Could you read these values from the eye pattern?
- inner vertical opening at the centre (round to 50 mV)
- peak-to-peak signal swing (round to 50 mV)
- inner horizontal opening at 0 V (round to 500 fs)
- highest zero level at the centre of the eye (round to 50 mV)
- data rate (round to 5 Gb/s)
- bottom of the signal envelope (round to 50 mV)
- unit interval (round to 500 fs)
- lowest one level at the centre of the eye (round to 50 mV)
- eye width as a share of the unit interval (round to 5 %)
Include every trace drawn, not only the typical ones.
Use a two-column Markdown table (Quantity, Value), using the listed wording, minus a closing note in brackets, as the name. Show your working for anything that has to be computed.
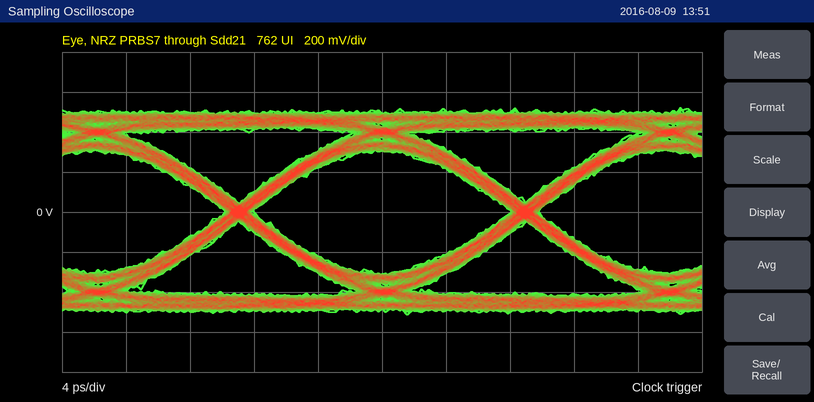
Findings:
| Quantity | Value |
|---|---|
| inner vertical opening at the centre | 600 mV |
| peak-to-peak signal swing | 1.05 V |
| inner horizontal opening at 0 V | 16.0 ps |
| highest zero level at the centre of the eye | -300 mV |
| data rate | 55 Gb/s |
| bottom of the signal envelope | -500 mV |
| unit interval | 18.0 ps |
| lowest one level at the centre of the eye | 300 mV |
| eye width as a share of the unit interval | 16.0 ps / 18.0 ps ≈ 88.9 %, so 90 % to the nearest 5 % |
